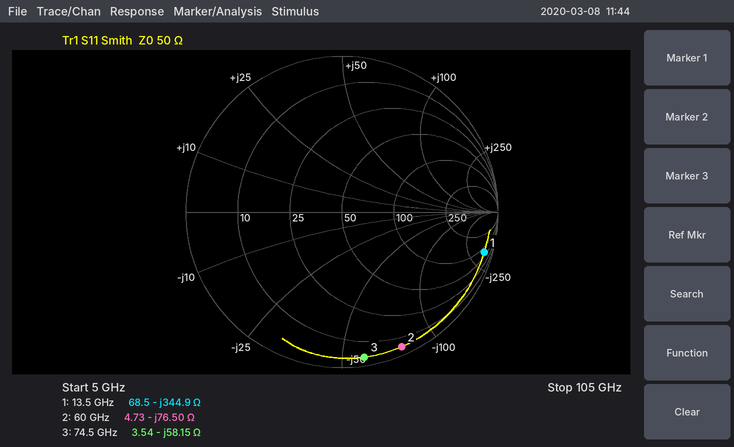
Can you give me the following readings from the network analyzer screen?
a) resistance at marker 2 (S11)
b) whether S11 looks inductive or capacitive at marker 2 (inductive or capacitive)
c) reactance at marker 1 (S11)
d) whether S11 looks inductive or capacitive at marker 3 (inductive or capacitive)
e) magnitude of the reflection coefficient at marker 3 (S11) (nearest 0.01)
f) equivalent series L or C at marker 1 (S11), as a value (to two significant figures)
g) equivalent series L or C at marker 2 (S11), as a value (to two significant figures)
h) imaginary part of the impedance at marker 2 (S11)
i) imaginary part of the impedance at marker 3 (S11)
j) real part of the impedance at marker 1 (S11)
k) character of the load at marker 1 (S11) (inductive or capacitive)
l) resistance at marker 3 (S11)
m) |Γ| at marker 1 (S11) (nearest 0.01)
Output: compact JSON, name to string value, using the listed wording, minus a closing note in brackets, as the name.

{"resistance at marker 2": "4.73 Ω", "whether S11 looks inductive or capacitive at marker 2": "capacitive", "reactance at marker 1": "-344.9 Ω", "whether S11 looks inductive or capacitive at marker 3": "capacitive", "magnitude of the reflection coefficient at marker 3 (S11)": "0.94", "equivalent series L or C at marker 1 (S11), as a value": "34 fF", "equivalent series L or C at marker 2 (S11), as a value": "35 fF", "imaginary part of the impedance at marker 2": "-76.50 Ω", "imaginary part of the impedance at marker 3": "-58.15 Ω", "real part of the impedance at marker 1": "68.5 Ω", "character of the load at marker 1 (S11)": "capacitive", "resistance at marker 3": "3.54 Ω", "|Γ| at marker 1 (S11)": "0.95"}
